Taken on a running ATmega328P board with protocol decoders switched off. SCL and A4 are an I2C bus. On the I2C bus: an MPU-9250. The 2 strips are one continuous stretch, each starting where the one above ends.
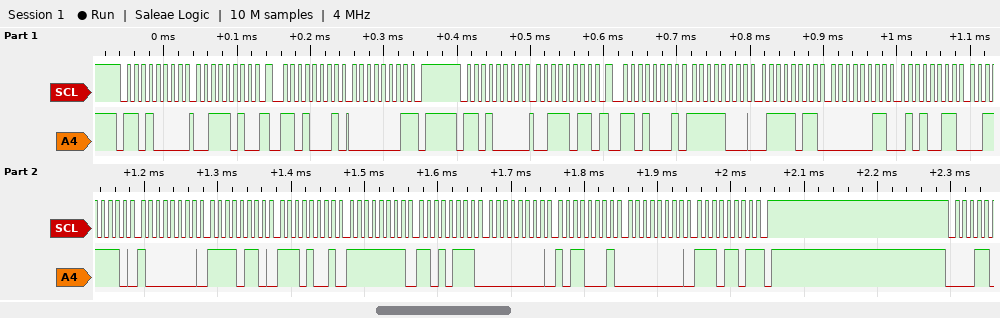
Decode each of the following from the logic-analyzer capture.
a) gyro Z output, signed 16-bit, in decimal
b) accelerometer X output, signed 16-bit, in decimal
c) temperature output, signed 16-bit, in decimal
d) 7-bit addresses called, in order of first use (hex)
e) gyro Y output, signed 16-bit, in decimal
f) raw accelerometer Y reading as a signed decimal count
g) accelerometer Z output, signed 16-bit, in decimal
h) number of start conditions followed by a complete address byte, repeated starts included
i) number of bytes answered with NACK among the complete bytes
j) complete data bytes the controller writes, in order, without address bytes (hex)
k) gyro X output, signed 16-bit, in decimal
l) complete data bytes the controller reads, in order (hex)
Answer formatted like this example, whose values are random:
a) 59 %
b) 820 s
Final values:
a) 237
b) -1925
c) -2327
d) 0x68
e) 177
f) 851
g) 16000
h) 4
i) 2
j) 3A 3B
k) -41
l) 01 F8 7B 03 53 3E 80 F6 E9 FF D7 00 B1 00 ED
